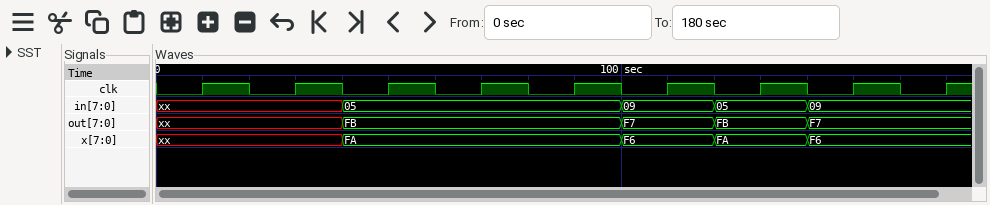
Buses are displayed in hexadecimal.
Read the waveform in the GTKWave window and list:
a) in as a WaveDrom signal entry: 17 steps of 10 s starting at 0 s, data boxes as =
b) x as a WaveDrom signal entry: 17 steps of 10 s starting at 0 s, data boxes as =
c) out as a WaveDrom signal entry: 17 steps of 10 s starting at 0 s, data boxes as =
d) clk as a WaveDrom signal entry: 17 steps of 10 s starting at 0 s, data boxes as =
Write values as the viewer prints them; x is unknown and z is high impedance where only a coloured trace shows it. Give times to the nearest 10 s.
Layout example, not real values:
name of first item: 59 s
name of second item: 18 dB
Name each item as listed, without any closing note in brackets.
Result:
in as a WaveDrom signal entry: 17 steps of 10 s starting at 0 s, data boxes as =: {name: 'in', wave: 'x...=.....=.=.=..', data: '05 09 05 09'}
x as a WaveDrom signal entry: 17 steps of 10 s starting at 0 s, data boxes as =: {name: 'x', wave: 'x...=.....=.=.=..', data: 'FA F6 FA F6'}
out as a WaveDrom signal entry: 17 steps of 10 s starting at 0 s, data boxes as =: {name: 'out', wave: 'x...=.....=.=.=..', data: 'FB F7 FB F7'}
clk as a WaveDrom signal entry: 17 steps of 10 s starting at 0 s, data boxes as =: {name: 'clk', wave: '01010101010101010'}
